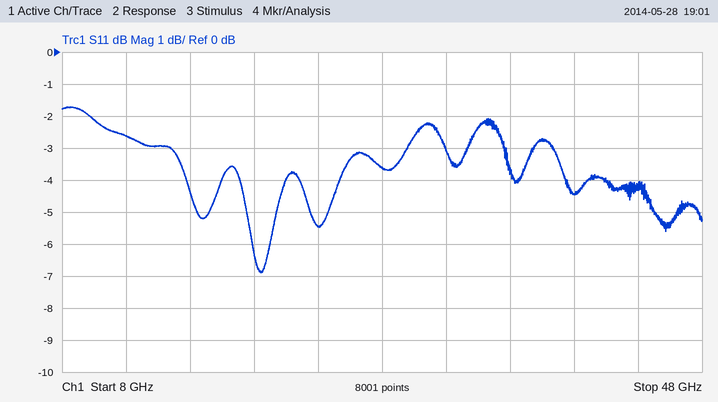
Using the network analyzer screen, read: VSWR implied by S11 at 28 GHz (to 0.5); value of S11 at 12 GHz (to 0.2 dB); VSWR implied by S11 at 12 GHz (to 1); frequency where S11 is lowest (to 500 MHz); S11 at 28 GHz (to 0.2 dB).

5.0
-2.6 dB
7
20.5 GHz
-3.6 dB
